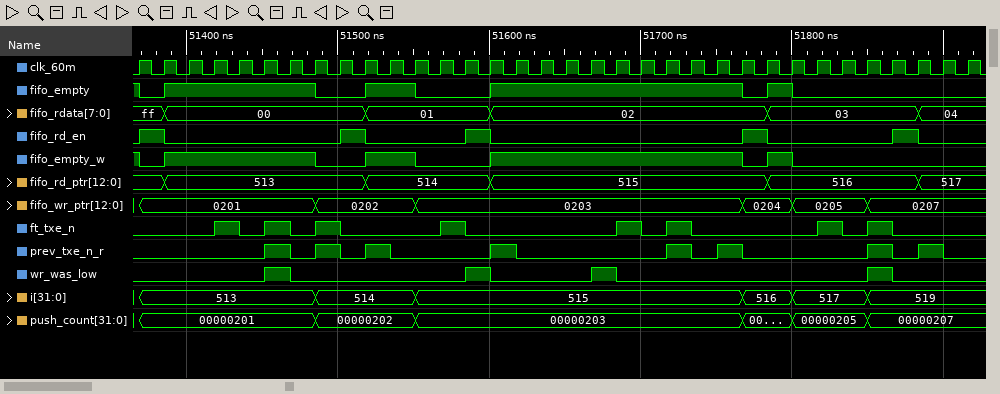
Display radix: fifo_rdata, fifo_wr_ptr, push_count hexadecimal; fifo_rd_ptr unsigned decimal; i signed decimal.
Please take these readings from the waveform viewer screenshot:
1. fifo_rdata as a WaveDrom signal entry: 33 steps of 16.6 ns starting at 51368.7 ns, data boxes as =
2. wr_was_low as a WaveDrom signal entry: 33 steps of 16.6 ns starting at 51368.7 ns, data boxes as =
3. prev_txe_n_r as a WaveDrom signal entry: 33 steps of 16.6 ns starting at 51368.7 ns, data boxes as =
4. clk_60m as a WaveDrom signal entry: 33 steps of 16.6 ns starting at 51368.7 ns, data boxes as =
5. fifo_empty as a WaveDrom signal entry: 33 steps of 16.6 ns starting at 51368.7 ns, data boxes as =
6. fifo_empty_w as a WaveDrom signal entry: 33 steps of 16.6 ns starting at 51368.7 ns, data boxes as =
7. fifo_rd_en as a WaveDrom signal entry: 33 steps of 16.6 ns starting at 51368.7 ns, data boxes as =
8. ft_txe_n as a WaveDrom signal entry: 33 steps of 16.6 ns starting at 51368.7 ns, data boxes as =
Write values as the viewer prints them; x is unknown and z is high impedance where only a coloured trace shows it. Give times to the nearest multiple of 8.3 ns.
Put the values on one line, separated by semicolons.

{name: 'fifo_rdata', wave: '==.......=....=..........=.....=.', data: 'ff 00 01 02 03 04'}; {name: 'wr_was_low', wave: '0....10......10...10.........10..'}; {name: 'prev_txe_n_r', wave: '0....101010...10.....1010....1010'}; {name: 'clk_60m', wave: 'p................................'}; {name: 'fifo_empty', wave: '01.....0.1.0..1.........010......'}; {name: 'fifo_empty_w', wave: '01.....0.1.0..1.........010......'}; {name: 'fifo_rd_en', wave: '10......10...10.........10....10.'}; {name: 'ft_txe_n', wave: '0..101010...10.....1010....1010..'}
